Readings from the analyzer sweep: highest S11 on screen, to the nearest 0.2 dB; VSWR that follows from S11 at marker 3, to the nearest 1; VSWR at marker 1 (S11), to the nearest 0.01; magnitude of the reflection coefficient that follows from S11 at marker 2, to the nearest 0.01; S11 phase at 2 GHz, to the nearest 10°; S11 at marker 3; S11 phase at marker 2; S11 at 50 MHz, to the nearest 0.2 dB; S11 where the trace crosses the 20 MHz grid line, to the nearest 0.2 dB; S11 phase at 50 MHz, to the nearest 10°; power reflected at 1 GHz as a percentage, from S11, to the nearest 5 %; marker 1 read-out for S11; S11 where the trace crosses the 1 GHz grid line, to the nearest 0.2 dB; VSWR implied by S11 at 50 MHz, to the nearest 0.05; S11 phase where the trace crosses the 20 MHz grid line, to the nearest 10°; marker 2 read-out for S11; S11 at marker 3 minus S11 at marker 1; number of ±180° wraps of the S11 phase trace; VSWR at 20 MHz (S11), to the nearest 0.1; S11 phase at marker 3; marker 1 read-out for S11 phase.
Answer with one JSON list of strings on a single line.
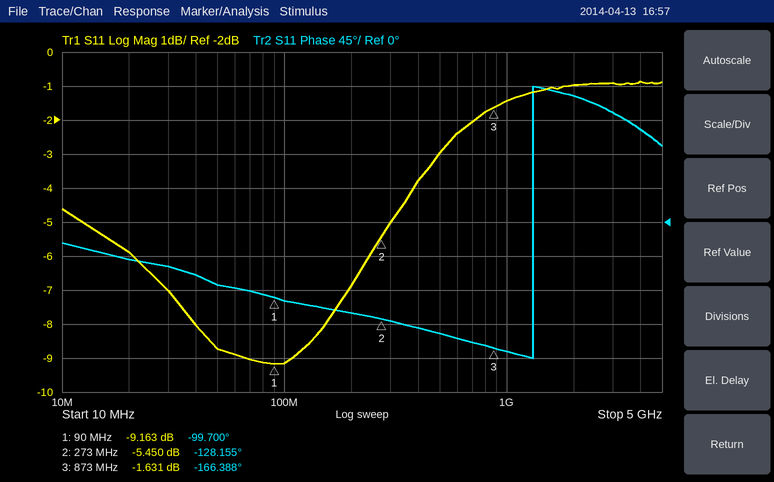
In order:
["-0.8 dB", "11", "2.07", "0.53", "170°", "-1.631 dB", "-128.155°", "-8.8 dB", "-5.8 dB", "-80°", "70 %", "-9.163 dB", "-1.4 dB", "2.15", "-50°", "-5.450 dB", "7.532 dB", "1", "3.1", "-166.388°", "-99.700°"]
